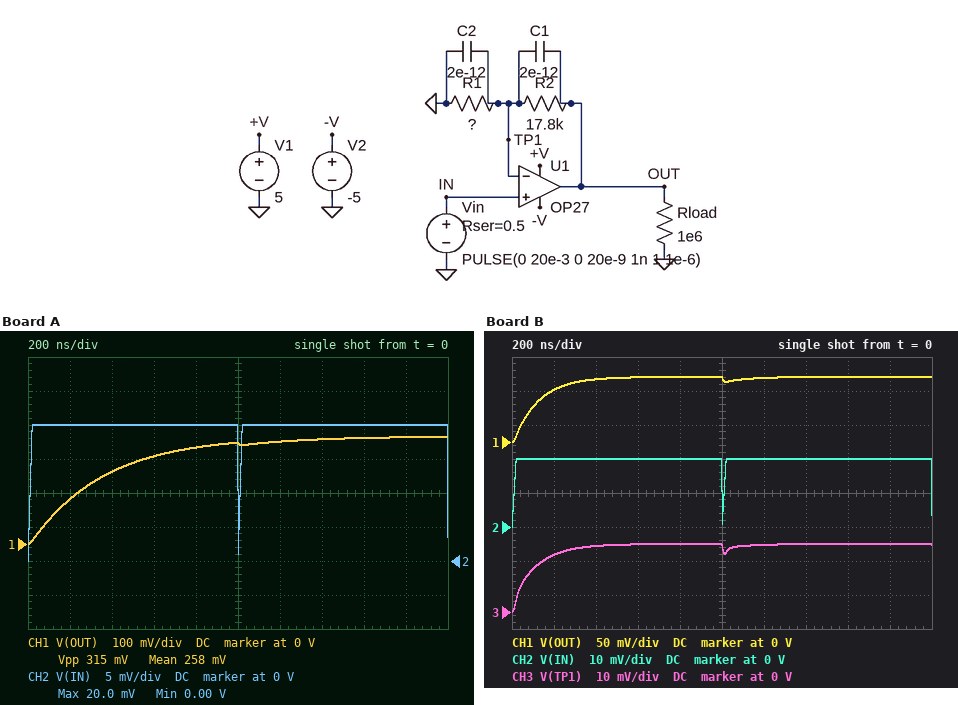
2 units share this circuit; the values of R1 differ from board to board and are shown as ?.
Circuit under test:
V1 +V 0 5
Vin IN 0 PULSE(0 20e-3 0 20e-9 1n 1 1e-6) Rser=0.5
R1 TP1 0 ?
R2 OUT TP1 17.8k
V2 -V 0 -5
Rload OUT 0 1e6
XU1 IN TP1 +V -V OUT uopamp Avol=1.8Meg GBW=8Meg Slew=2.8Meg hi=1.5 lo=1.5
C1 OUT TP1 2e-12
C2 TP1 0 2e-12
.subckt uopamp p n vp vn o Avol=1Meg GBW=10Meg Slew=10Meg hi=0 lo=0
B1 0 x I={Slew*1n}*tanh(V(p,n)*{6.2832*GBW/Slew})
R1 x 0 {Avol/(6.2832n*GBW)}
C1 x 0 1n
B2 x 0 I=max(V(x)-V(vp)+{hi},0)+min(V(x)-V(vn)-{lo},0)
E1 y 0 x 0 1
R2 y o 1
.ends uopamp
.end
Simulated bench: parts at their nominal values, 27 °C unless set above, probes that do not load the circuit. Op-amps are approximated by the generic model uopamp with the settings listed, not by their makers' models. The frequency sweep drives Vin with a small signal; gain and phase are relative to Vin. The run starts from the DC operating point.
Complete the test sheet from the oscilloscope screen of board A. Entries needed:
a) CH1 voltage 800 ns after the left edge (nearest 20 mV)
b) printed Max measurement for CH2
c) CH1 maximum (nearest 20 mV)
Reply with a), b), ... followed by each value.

a) 280 mV
b) 20.0 mV
c) 320 mV
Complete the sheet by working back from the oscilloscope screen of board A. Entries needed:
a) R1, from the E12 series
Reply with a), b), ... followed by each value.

a) 1.2 kΩ
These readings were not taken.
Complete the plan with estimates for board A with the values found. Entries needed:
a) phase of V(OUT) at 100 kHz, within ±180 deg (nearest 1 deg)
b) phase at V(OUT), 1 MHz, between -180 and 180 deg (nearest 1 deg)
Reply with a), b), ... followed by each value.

a) -12 deg
b) -65 deg
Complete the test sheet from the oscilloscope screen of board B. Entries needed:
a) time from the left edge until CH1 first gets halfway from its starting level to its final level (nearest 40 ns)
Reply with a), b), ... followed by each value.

a) 80 ns
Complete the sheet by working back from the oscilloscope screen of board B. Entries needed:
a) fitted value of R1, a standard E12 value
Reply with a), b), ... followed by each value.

a) 4.7 kΩ
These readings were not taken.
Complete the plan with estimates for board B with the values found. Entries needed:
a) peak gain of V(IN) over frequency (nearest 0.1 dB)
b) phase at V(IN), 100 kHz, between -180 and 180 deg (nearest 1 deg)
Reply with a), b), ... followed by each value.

a) 0 dB
b) 0 deg
